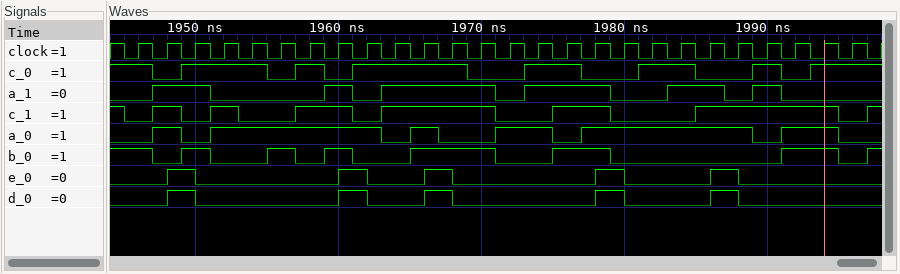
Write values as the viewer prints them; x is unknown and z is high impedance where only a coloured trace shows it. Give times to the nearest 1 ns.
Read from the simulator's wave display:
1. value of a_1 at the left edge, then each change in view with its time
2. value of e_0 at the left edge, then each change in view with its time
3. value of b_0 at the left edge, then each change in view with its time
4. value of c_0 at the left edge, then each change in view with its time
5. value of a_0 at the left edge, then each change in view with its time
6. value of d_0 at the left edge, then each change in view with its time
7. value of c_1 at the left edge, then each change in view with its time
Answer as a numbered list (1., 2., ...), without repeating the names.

1. 0, 1 at 1947 ns, 0 at 1951 ns, 1 at 1959 ns, 0 at 1961 ns, 1 at 1963 ns, 0 at 1971 ns, 1 at 1973 ns, 0 at 1979 ns, 1 at 1983 ns, 0 at 1987 ns, 1 at 1989 ns, 0 at 1991 ns
2. 0, 1 at 1948 ns, 0 at 1950 ns, 1 at 1960 ns, 0 at 1962 ns, 1 at 1966 ns, 0 at 1968 ns, 1 at 1978 ns, 0 at 1980 ns, 1 at 1986 ns, 0 at 1988 ns
3. 1, 0 at 1947 ns, 1 at 1949 ns, 0 at 1951 ns, 1 at 1955 ns, 0 at 1957 ns, 1 at 1959 ns, 0 at 1961 ns, 1 at 1965 ns, 0 at 1971 ns, 1 at 1975 ns, 0 at 1979 ns, 1 at 1991 ns, 0 at 1995 ns, 1 at 1997 ns
4. 1, 0 at 1947 ns, 1 at 1949 ns, 0 at 1955 ns, 1 at 1957 ns, 0 at 1959 ns, 1 at 1961 ns, 0 at 1969 ns, 1 at 1973 ns, 0 at 1977 ns, 1 at 1981 ns, 0 at 1985 ns, 1 at 1989 ns, 0 at 1991 ns, 1 at 1993 ns
5. 0, 1 at 1947 ns, 0 at 1949 ns, 1 at 1951 ns, 0 at 1963 ns, 1 at 1965 ns, 0 at 1967 ns, 1 at 1971 ns, 0 at 1975 ns, 1 at 1977 ns, 0 at 1989 ns, 1 at 1991 ns, 0 at 1995 ns
6. 0, 1 at 1948 ns, 0 at 1950 ns, 1 at 1960 ns, 0 at 1962 ns, 1 at 1966 ns, 0 at 1968 ns, 1 at 1978 ns, 0 at 1980 ns, 1 at 1986 ns, 0 at 1988 ns
7. 1, 0 at 1945 ns, 1 at 1947 ns, 0 at 1949 ns, 1 at 1951 ns, 0 at 1953 ns, 1 at 1957 ns, 0 at 1961 ns, 1 at 1963 ns, 0 at 1971 ns, 1 at 1975 ns, 0 at 1979 ns, 1 at 1985 ns, 0 at 1995 ns, 1 at 1997 ns
